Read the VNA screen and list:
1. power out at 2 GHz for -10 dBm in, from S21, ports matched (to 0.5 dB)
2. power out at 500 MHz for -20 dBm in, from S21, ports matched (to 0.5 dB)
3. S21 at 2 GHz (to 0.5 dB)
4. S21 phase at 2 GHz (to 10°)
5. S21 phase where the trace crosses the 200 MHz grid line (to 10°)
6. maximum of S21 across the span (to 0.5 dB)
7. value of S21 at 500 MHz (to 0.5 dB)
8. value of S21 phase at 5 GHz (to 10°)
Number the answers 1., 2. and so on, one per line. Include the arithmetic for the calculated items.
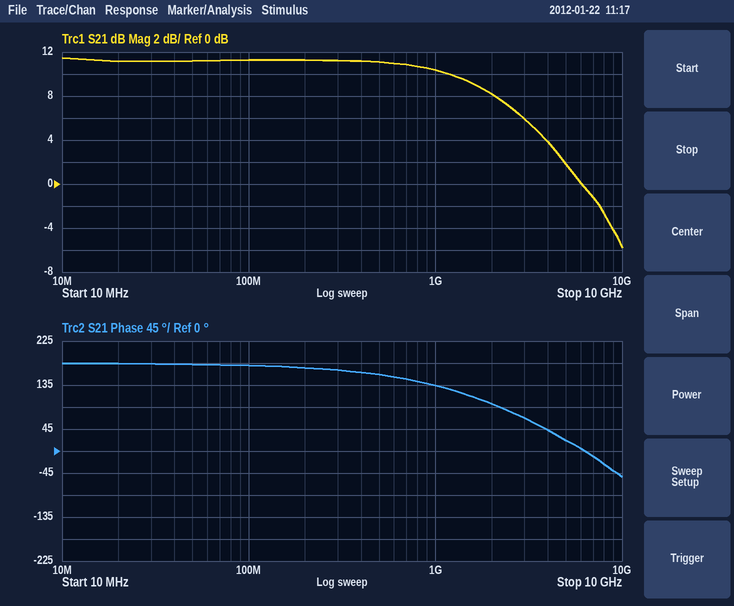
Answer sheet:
1. -10 dBm + (8.0 dB) = -2.0 dBm
2. -20 dBm + (11.0 dB) = -9.0 dBm
3. 8.0 dB
4. 100°
5. 170°
6. 11.5 dB
7. 11.0 dB
8. 20°
